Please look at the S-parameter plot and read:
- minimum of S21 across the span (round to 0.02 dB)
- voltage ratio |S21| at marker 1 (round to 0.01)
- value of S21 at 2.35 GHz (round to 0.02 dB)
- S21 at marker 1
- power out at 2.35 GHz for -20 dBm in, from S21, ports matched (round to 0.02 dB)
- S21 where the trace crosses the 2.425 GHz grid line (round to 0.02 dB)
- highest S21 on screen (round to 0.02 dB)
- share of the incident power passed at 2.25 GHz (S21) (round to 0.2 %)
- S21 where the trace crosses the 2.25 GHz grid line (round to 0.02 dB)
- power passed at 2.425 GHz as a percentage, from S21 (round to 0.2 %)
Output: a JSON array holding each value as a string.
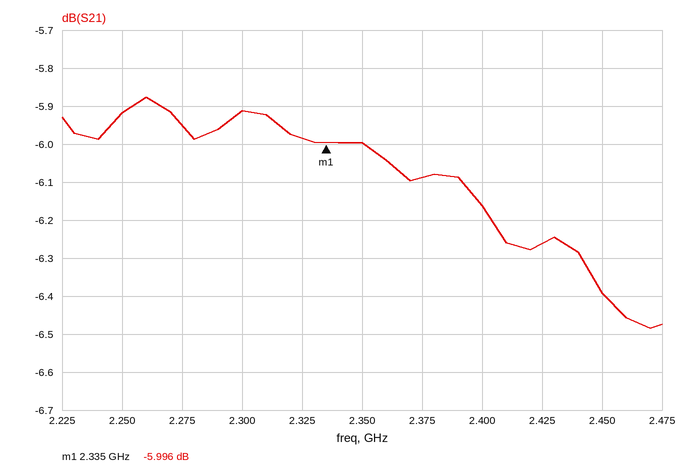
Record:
["-6.48 dB", "0.50", "-6.00 dB", "-5.996 dB", "-26.00 dBm", "-6.26 dB", "-5.88 dB", "25.6 %", "-5.92 dB", "23.6 %"]
